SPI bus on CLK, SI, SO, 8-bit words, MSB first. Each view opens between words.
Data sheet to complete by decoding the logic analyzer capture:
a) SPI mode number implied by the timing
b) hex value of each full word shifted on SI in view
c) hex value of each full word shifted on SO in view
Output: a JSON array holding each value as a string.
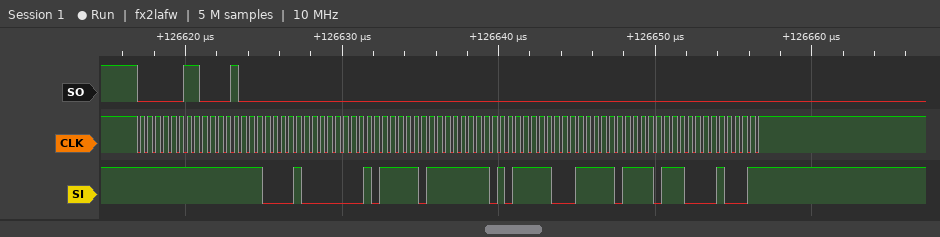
["3", "FF, FF, 08, 05, F7, FA, F8, FB, DC, 23", "03, 08, 00, 00, 00, 00, 00, 00, 00, 00"]
